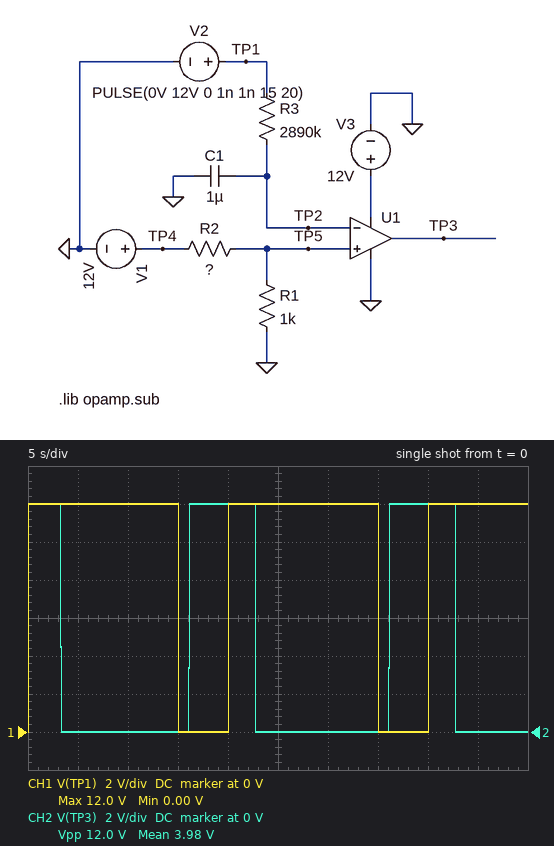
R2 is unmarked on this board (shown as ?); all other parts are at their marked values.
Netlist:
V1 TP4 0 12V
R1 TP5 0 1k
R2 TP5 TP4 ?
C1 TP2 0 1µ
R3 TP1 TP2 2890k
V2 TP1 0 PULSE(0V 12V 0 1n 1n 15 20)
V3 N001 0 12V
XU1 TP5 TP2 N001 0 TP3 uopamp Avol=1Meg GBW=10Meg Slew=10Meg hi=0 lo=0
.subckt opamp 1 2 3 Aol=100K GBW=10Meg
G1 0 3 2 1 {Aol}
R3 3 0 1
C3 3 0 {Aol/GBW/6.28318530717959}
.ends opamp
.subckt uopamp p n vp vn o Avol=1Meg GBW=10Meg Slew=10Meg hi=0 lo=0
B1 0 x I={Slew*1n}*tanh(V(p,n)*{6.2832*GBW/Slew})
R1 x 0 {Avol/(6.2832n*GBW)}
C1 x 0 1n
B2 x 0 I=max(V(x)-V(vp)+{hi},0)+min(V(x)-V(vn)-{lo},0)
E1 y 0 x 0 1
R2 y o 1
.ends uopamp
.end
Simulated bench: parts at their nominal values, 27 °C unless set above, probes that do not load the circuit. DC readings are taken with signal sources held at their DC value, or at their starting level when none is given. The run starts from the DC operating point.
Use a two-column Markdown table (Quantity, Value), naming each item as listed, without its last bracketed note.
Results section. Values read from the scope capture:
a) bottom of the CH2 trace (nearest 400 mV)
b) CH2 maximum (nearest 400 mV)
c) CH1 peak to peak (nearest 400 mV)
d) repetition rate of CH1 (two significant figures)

| Quantity | Value |
|---|---|
| bottom of the CH2 trace | 0 V |
| CH2 maximum | 12.0 V |
| CH1 peak to peak | 12.0 V |
| repetition rate of CH1 | 50 mHz |
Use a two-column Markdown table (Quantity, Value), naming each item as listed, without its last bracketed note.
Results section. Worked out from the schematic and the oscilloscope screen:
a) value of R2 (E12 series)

| Quantity | Value |
|---|---|
| value of R2 | 470 Ω |
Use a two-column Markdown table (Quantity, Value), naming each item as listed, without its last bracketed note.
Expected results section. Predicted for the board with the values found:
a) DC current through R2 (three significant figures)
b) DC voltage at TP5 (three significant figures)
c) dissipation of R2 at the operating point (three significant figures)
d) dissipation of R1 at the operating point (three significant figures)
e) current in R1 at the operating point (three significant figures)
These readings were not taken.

| Quantity | Value |
|---|---|
| DC current through R2 | 8.16 mA |
| DC voltage at TP5 | 8.16 V |
| dissipation of R2 at the operating point | 31.3 mW |
| dissipation of R1 at the operating point | 66.6 mW |
| current in R1 at the operating point | 8.16 mA |
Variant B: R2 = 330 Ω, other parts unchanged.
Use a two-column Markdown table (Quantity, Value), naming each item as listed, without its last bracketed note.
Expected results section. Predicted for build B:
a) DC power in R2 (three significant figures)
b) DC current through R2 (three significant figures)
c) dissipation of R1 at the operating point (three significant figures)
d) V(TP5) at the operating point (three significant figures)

| Quantity | Value |
|---|---|
| DC power in R2 | 26.9 mW |
| DC current through R2 | 9.02 mA |
| dissipation of R1 at the operating point | 81.4 mW |
| V(TP5) at the operating point | 9.02 V |
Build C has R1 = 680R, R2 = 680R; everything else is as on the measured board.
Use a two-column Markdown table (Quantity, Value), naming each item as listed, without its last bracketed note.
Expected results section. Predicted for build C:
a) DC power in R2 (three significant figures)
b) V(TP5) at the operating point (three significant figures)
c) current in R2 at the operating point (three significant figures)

| Quantity | Value |
|---|---|
| DC power in R2 | 52.9 mW |
| V(TP5) at the operating point | 6.00 V |
| current in R2 at the operating point | 8.82 mA |
